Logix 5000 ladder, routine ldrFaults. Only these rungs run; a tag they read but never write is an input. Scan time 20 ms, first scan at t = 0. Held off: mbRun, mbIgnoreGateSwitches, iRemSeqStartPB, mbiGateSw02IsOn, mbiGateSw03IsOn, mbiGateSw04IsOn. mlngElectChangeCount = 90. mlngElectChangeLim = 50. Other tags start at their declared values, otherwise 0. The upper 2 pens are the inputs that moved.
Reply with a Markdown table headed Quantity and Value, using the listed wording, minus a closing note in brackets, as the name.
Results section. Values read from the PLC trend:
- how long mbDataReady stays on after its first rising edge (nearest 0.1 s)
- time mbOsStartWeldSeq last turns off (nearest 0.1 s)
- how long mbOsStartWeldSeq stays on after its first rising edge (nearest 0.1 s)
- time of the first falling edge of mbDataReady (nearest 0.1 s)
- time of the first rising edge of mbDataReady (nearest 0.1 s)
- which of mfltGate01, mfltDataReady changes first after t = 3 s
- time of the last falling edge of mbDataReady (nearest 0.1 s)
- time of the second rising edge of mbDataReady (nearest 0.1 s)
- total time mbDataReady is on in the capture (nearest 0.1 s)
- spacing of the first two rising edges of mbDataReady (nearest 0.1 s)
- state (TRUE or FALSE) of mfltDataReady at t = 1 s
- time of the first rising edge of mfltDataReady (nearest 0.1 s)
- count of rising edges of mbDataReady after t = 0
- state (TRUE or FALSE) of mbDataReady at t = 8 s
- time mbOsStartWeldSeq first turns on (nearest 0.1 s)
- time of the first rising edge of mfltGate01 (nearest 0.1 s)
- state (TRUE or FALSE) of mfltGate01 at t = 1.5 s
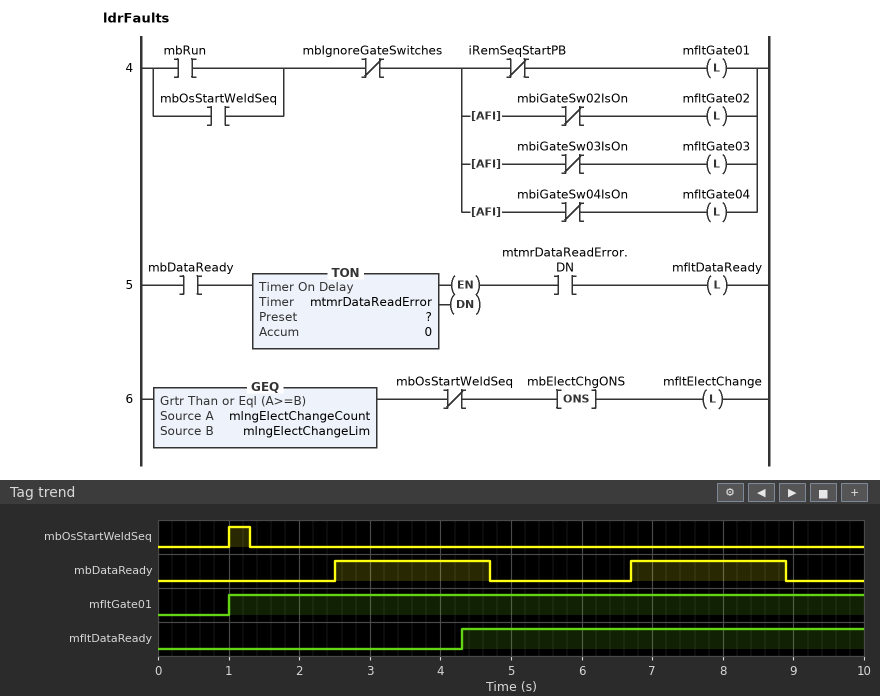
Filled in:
| Quantity | Value |
|---|---|
| how long mbDataReady stays on after its first rising edge | 2.2 s |
| time mbOsStartWeldSeq last turns off | 1.3 s |
| how long mbOsStartWeldSeq stays on after its first rising edge | 0.3 s |
| time of the first falling edge of mbDataReady | 4.7 s |
| time of the first rising edge of mbDataReady | 2.5 s |
| which of mfltGate01, mfltDataReady changes first after t = 3 s | mfltDataReady |
| time of the last falling edge of mbDataReady | 8.9 s |
| time of the second rising edge of mbDataReady | 6.7 s |
| total time mbDataReady is on in the capture | 4.4 s |
| spacing of the first two rising edges of mbDataReady | 4.2 s |
| state (TRUE or FALSE) of mfltDataReady at t = 1 s | FALSE |
| time of the first rising edge of mfltDataReady | 4.3 s |
| count of rising edges of mbDataReady after t = 0 | 2 |
| state (TRUE or FALSE) of mbDataReady at t = 8 s | TRUE |
| time mbOsStartWeldSeq first turns on | 1.0 s |
| time of the first rising edge of mfltGate01 | 1.0 s |
| state (TRUE or FALSE) of mfltGate01 at t = 1.5 s | TRUE |
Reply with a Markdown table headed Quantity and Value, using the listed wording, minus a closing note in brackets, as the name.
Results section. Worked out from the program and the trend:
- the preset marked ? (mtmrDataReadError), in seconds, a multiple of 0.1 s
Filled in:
| Quantity | Value |
|---|---|
| the preset marked ? (mtmrDataReadError), in seconds, a multiple of 0.1 s | 1.8 s |
